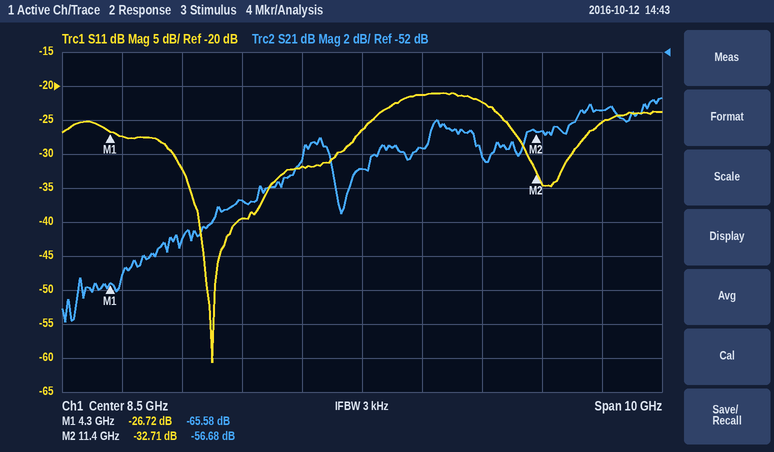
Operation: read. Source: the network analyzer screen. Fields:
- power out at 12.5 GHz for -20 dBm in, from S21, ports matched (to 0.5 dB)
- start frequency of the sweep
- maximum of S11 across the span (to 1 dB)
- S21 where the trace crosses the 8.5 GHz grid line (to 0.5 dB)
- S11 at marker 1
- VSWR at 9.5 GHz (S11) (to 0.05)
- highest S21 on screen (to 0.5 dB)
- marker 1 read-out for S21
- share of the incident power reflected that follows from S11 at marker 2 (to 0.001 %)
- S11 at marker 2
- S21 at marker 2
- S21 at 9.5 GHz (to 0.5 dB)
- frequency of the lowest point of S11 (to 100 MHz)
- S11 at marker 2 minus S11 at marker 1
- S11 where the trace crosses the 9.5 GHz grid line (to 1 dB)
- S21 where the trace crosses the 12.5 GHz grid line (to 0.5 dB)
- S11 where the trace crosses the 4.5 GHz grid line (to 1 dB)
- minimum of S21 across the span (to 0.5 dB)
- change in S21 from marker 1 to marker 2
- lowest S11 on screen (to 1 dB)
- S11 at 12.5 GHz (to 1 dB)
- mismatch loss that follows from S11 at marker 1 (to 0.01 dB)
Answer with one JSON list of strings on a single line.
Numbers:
["-75.5 dBm", "3.5 GHz", "-21 dB", "-59.0 dB", "-26.72 dB", "1.20", "-54.5 dB", "-65.58 dB", "0.054 %", "-32.71 dB", "-56.68 dB", "-57.5 dB", "6.0 GHz", "-5.99 dB", "-21 dB", "-55.5 dB", "-27 dB", "-68.0 dB", "8.90 dB", "-61 dB", "-25 dB", "0.01 dB"]
